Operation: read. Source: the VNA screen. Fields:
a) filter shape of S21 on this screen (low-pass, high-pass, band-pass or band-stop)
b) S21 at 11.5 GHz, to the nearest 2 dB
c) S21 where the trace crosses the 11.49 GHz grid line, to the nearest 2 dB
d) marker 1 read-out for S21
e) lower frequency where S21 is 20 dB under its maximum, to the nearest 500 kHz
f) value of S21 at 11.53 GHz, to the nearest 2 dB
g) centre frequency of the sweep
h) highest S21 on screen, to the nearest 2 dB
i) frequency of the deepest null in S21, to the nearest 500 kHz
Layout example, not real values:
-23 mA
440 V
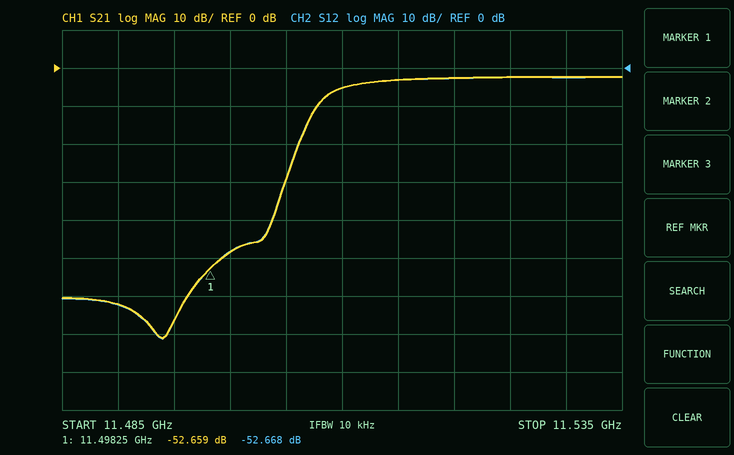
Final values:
high-pass
-48 dB
-62 dB
-52.659 dB
11.5060 GHz
-2 dB
11.51 GHz
-2 dB
11.4940 GHz
